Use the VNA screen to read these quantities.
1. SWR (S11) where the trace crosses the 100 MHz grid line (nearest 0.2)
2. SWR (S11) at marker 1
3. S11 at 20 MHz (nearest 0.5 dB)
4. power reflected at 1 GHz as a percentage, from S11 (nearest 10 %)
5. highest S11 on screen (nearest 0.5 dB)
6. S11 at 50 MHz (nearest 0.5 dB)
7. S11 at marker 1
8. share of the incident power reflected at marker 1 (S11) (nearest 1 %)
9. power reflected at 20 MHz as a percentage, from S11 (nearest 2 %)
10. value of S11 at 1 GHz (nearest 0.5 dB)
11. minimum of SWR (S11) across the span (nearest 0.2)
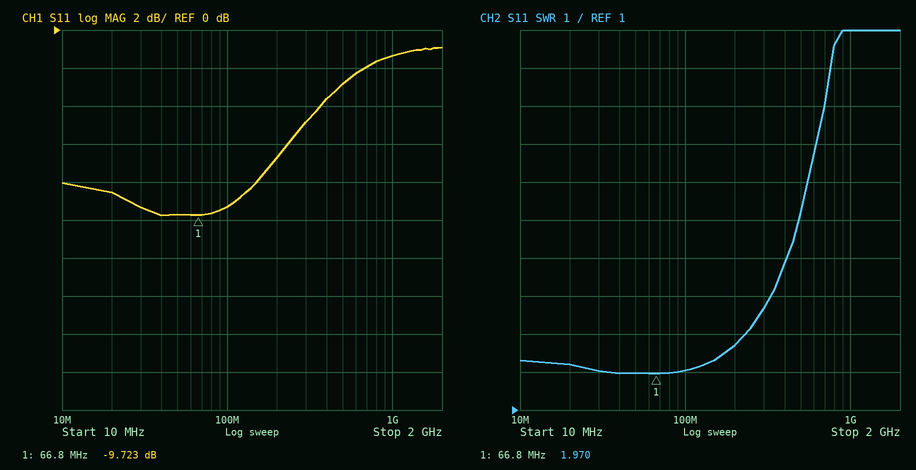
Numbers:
2.0
1.970
-8.5 dB
70 %
-1.0 dB
-9.5 dB
-9.723 dB
11 %
14 %
-1.5 dB
2.0
